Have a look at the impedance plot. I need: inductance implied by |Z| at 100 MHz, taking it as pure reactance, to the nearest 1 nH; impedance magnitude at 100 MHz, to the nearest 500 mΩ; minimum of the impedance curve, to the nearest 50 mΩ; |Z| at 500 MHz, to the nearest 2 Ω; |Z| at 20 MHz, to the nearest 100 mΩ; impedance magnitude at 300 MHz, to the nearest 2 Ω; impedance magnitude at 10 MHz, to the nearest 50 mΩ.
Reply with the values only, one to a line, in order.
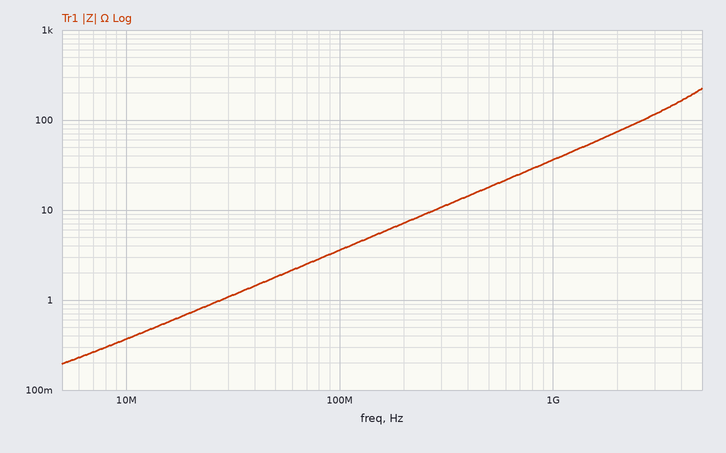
6 nH
3.5 Ω
200 mΩ
18 Ω
700 mΩ
10 Ω
350 mΩ
